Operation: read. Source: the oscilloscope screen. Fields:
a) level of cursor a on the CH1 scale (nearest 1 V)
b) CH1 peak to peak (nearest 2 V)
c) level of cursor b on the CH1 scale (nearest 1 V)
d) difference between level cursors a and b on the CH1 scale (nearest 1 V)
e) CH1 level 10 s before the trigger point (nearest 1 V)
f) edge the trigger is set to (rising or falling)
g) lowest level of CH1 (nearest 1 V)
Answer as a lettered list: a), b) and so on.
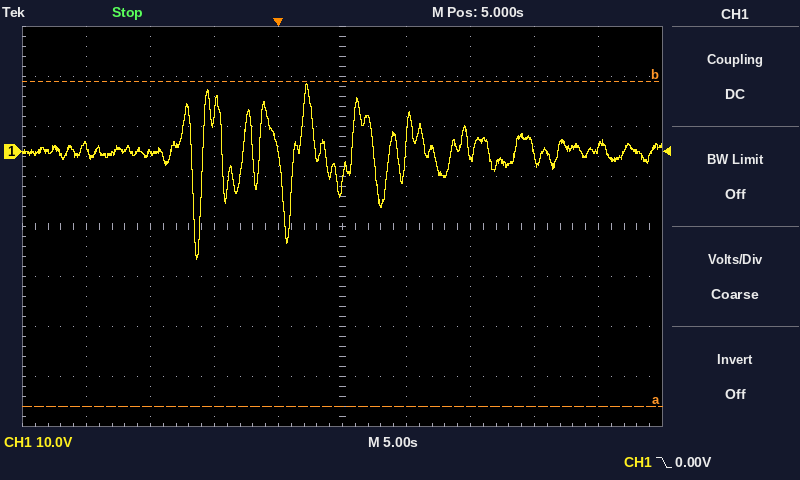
a) -51 V
b) 36 V
c) 14 V
d) 65 V
e) 0 V
f) falling
g) -22 V
